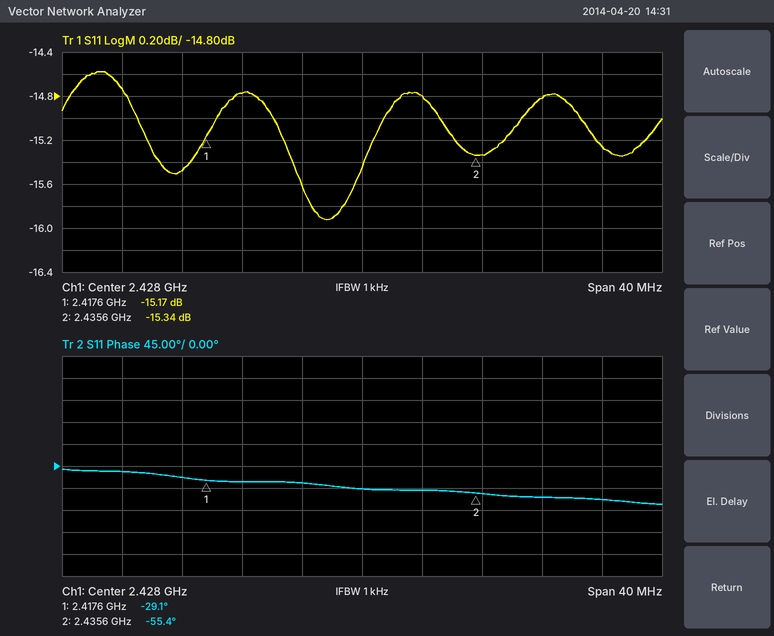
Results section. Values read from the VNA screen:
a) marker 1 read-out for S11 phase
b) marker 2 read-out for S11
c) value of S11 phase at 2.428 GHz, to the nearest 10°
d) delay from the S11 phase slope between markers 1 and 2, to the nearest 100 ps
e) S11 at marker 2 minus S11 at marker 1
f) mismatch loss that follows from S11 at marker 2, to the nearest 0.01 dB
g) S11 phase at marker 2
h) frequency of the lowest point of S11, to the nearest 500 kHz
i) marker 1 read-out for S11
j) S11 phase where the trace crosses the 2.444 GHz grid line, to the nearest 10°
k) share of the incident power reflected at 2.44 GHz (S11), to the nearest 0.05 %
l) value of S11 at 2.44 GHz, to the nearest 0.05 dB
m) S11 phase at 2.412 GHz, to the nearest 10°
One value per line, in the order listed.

-29.1°
-15.34 dB
-50°
4.1 ns
-0.17 dB
0.13 dB
-55.4°
2.4255 GHz
-15.17 dB
-70°
3.30 %
-14.80 dB
-10°
